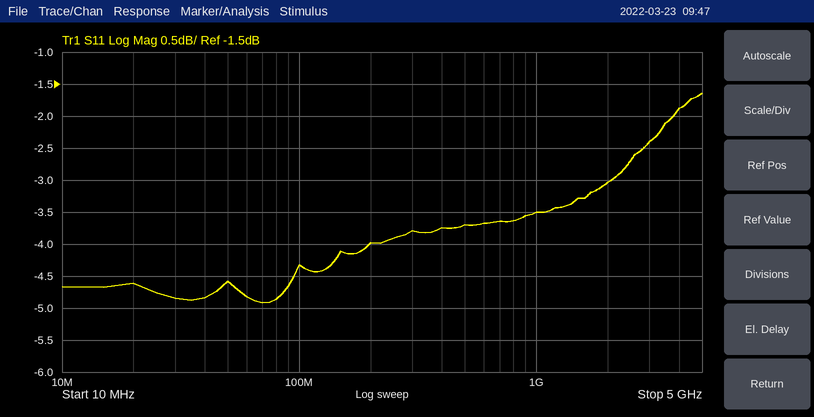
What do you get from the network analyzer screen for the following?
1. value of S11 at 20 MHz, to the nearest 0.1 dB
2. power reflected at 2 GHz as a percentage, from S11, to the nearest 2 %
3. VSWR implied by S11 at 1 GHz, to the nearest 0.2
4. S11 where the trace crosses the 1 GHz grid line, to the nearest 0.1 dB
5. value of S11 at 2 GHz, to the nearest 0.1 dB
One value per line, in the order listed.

-4.6 dB
50 %
5.0
-3.5 dB
-3.0 dB
